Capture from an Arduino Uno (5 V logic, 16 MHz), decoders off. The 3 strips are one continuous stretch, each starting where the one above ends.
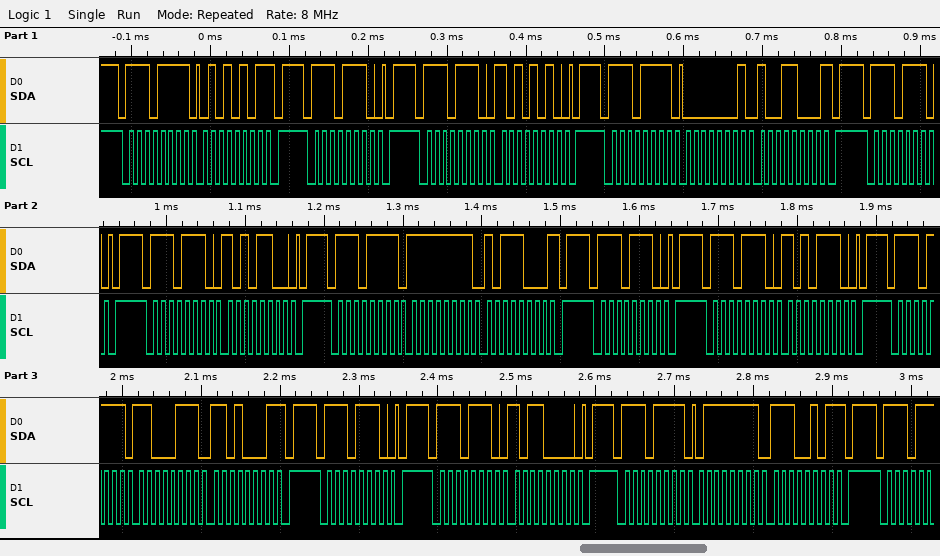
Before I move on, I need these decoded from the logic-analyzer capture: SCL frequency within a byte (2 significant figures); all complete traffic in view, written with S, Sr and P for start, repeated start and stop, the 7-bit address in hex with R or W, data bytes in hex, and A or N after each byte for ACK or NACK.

100 kHz
S 77R A 55 N P S 77W A P S 77W A AA A P S 77R A 01 A 98 N P S 77W A P S 77W A AC A P S 77R A FF A B8 N P S 77W A P S 77W A AE A P S 77R A C7 A D1 N P S 77W A P S 77W A B0 A P S 77R A 7F A E5 N P
